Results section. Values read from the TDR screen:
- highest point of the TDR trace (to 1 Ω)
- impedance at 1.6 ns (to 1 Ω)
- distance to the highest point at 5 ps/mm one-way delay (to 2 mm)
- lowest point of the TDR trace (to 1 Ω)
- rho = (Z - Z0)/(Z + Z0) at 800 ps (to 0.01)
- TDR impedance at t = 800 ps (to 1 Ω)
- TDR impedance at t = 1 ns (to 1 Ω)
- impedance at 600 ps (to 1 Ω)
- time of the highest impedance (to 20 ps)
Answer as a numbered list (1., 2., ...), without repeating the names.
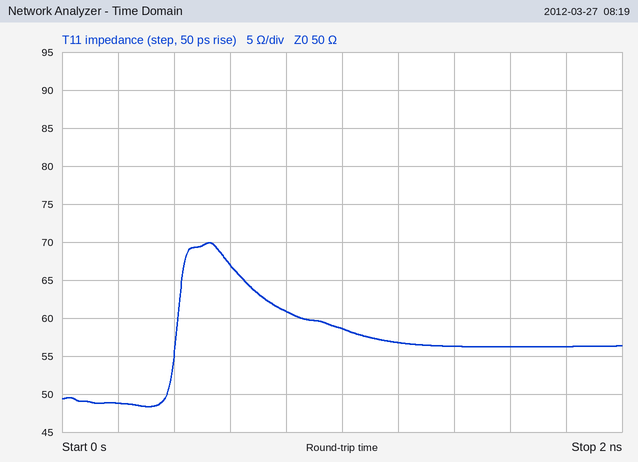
1. 70 Ω
2. 56 Ω
3. 52 mm
4. 48 Ω
5. +0.10
6. 61 Ω
7. 59 Ω
8. 67 Ω
9. 520 ps
